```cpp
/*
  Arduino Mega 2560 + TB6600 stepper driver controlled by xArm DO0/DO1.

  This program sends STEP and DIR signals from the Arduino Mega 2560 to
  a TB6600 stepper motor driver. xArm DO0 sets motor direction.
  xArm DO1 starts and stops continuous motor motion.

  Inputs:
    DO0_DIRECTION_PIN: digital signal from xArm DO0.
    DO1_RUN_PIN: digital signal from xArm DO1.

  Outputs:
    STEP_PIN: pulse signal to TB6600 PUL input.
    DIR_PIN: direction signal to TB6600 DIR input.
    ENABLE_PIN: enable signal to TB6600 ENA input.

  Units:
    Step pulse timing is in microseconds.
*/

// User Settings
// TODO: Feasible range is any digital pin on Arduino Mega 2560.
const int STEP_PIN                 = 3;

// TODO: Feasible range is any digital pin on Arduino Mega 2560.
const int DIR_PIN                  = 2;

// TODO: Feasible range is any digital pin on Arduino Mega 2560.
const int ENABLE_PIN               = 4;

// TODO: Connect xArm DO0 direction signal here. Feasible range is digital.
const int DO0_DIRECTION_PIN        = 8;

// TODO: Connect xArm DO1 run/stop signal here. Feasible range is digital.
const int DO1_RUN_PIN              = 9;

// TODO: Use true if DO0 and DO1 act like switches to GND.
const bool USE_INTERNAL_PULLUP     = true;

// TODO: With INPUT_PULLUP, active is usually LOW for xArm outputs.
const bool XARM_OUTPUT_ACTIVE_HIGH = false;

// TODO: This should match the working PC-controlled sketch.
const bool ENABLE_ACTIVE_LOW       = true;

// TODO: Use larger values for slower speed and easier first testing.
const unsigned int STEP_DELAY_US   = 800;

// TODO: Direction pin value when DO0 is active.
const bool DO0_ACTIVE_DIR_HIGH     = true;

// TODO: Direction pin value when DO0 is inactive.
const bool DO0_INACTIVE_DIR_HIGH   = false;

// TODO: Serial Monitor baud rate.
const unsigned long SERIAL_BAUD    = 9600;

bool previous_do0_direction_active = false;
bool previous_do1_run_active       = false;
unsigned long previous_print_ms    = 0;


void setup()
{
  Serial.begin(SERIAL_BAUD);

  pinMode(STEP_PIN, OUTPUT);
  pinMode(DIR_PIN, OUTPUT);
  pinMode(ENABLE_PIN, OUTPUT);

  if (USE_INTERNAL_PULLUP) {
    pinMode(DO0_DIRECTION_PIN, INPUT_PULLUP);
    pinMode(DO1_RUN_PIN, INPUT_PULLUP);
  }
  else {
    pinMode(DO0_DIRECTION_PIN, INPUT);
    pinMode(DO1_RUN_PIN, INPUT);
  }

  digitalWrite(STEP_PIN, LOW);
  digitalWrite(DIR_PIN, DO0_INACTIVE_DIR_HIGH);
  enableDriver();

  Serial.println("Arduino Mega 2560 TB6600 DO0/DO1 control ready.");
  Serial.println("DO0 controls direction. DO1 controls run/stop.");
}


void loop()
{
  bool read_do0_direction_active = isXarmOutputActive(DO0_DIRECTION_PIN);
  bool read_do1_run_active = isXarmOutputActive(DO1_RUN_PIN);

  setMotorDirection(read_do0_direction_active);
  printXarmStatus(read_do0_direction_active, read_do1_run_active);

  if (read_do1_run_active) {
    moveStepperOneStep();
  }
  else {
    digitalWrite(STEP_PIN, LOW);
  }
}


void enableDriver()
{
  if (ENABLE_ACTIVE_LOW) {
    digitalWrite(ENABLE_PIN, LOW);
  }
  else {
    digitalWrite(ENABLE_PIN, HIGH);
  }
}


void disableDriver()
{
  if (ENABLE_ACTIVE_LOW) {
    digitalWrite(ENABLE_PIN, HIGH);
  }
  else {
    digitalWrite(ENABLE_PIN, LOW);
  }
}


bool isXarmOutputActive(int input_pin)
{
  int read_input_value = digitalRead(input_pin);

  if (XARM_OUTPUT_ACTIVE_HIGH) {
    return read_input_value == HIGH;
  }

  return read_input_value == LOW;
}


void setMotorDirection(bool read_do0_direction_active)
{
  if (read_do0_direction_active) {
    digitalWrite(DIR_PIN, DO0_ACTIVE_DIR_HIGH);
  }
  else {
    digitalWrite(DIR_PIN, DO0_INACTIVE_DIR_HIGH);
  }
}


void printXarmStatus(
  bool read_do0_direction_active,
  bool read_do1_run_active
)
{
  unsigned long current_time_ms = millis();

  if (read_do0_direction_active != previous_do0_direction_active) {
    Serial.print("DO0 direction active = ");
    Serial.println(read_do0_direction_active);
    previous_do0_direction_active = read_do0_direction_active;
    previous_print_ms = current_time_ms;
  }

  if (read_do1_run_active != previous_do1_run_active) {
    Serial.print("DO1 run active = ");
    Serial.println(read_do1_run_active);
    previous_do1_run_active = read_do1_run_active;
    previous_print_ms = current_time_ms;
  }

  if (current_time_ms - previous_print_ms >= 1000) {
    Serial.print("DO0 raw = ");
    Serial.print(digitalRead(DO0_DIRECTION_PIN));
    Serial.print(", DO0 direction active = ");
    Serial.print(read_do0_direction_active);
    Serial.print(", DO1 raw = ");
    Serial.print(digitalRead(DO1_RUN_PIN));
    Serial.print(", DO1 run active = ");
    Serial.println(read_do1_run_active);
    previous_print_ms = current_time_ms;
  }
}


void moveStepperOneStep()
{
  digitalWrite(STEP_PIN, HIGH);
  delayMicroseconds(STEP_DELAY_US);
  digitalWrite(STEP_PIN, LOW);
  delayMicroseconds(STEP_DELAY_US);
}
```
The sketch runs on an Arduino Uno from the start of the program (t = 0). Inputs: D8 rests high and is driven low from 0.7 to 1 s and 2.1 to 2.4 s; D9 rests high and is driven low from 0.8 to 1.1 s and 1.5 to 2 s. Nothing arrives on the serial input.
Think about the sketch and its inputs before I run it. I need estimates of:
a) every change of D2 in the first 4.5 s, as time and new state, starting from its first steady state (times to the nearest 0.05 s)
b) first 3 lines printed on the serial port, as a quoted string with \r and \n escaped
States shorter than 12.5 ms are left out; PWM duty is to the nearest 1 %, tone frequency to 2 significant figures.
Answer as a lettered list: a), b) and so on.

a) 0 s low; 0.7 s high; 1 s low; 2.1 s high; 2.4 s low
b) "Arduino Mega 2560 TB6600 DO0/DO1 control ready.\r\nDO0 controls direction. DO1 controls run/stop.\r\nDO0 direction active = 1\r\n"
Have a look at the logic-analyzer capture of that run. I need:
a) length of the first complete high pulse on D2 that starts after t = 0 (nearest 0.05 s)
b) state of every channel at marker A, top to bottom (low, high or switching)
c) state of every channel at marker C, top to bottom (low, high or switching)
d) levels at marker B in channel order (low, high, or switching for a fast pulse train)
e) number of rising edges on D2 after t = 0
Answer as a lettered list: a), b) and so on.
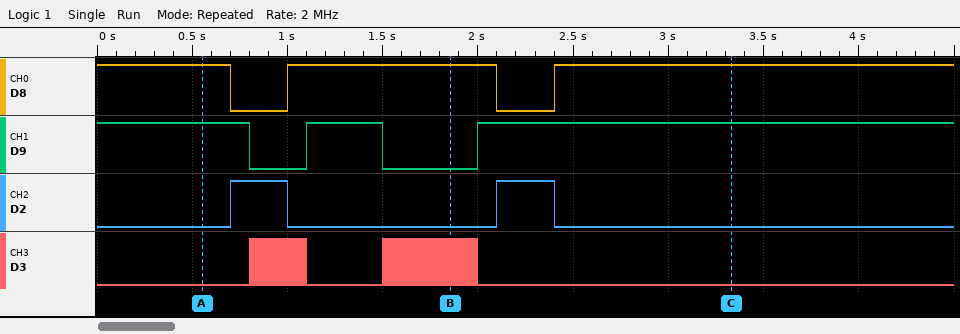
a) 0.30 s
b) D8 high, D9 high, D2 low, D3 low
c) D8 high, D9 high, D2 low, D3 low
d) D8 high, D9 low, D2 low, D3 switching
e) 2
